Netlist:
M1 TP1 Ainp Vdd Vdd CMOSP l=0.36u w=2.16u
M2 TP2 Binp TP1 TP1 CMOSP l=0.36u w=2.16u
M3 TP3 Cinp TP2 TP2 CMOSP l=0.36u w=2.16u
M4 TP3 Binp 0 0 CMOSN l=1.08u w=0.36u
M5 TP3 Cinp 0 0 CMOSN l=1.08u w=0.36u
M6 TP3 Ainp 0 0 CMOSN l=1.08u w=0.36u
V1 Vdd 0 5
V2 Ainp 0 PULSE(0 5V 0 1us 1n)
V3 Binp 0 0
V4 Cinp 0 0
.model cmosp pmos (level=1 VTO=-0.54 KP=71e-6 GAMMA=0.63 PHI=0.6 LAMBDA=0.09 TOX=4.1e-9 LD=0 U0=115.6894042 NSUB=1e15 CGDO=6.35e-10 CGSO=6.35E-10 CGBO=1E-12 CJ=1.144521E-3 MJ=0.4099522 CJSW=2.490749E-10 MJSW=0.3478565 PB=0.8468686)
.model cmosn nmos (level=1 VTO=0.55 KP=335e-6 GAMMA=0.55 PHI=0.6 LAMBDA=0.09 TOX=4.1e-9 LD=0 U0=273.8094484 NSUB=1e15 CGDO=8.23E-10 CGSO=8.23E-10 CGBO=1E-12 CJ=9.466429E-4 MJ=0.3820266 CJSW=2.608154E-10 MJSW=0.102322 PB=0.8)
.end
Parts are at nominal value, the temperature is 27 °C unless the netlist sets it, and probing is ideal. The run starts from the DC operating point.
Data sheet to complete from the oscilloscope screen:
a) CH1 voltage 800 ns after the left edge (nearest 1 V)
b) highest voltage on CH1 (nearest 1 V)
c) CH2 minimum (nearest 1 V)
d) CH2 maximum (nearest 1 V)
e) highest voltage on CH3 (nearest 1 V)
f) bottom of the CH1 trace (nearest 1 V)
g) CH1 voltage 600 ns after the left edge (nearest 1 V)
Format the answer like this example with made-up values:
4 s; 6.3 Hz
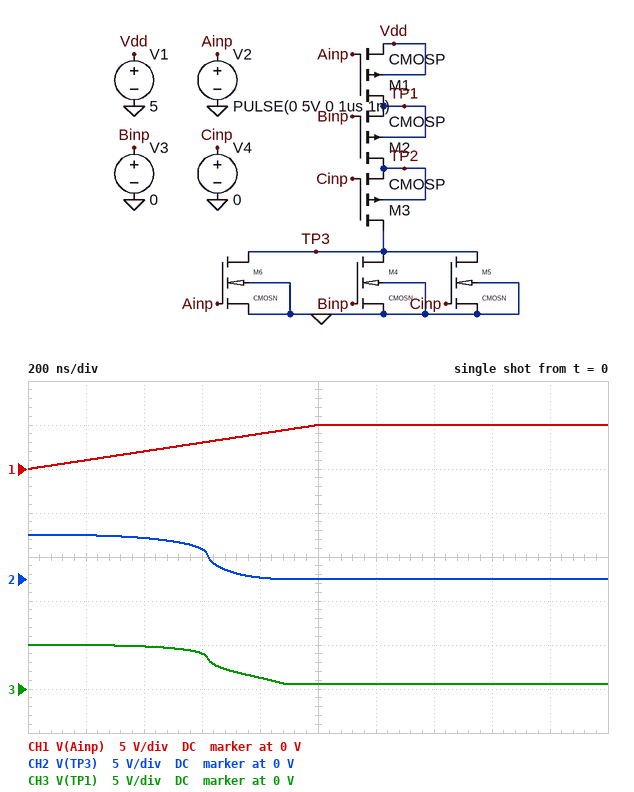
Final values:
4 V; 5 V; 0 V; 5 V; 5 V; 0 V; 3 V
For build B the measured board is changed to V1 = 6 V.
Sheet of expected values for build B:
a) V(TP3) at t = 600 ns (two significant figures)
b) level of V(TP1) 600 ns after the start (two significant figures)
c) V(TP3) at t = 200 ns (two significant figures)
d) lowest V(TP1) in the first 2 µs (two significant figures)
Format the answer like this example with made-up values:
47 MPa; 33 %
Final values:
5.0 V; 5.5 V; 6.0 V; 1.3 V
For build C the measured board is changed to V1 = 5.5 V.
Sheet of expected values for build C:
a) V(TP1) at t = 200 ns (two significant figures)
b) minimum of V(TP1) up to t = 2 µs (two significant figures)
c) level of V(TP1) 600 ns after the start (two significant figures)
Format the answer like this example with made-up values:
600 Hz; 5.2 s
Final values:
5.5 V; 540 mV; 4.9 V
